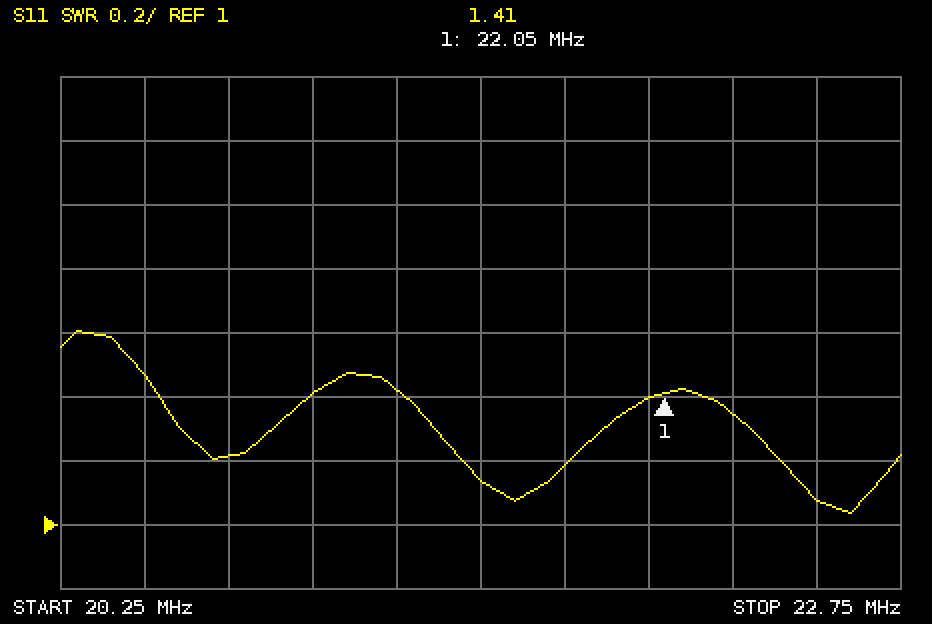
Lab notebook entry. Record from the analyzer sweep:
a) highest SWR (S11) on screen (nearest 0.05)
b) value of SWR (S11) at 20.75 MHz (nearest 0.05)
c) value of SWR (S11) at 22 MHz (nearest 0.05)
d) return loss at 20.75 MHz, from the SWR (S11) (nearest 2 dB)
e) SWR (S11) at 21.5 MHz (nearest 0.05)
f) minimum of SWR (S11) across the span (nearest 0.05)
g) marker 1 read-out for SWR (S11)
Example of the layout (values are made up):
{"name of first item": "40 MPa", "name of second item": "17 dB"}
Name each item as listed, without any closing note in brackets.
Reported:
{"highest SWR (S11) on screen": "1.60", "value of SWR (S11) at 20.75 MHz": "1.20", "value of SWR (S11) at 22 MHz": "1.40", "return loss at 20.75 MHz, from the SWR (S11)": "20 dB", "SWR (S11) at 21.5 MHz": "1.15", "minimum of SWR (S11) across the span": "1.05", "marker 1 read-out for SWR": "1.41"}
